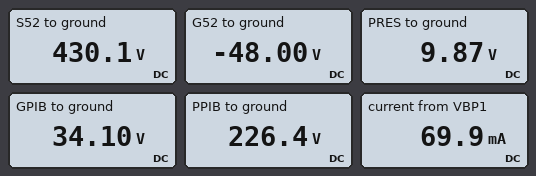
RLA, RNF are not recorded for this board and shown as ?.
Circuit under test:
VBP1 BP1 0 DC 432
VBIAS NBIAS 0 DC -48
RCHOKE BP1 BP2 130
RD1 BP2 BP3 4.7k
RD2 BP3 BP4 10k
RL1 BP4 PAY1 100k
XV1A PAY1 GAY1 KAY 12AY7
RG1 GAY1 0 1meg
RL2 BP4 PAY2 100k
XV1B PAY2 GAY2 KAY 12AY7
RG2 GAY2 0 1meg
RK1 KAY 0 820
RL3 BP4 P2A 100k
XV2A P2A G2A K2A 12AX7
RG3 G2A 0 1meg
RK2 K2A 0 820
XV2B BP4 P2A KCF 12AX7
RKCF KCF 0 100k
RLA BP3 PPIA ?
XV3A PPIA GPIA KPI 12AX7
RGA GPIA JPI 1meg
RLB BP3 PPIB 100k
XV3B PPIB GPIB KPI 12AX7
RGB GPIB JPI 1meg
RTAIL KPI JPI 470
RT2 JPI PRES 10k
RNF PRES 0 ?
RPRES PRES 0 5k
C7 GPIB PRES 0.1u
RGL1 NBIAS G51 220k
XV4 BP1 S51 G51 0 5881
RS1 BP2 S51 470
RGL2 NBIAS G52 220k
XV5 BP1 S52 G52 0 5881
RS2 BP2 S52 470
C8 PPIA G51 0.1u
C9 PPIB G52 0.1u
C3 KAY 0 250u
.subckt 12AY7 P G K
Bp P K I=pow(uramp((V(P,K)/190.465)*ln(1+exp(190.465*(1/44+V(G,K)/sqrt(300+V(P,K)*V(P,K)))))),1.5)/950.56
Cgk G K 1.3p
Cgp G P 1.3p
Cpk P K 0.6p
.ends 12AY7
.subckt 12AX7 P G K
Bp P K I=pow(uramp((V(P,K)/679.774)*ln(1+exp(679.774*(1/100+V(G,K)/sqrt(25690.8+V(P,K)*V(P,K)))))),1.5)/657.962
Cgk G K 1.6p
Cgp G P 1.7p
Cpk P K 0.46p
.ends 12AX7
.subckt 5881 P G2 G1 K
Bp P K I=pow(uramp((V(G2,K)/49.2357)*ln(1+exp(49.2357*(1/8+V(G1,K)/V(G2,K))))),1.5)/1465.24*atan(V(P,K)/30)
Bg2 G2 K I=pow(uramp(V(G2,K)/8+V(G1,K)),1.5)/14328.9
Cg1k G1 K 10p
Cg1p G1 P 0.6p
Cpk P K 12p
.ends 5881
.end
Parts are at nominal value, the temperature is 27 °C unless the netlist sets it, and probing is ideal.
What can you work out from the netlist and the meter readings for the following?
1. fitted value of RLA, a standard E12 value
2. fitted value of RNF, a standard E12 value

270 kΩ
22 kΩ
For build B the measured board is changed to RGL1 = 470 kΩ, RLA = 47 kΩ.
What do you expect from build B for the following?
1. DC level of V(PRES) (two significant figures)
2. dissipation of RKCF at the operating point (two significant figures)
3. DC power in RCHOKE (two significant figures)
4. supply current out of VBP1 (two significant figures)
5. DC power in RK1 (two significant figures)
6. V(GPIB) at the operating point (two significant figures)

13 V
330 mW
17 mW
71 mA
8.1 mW
46 V
